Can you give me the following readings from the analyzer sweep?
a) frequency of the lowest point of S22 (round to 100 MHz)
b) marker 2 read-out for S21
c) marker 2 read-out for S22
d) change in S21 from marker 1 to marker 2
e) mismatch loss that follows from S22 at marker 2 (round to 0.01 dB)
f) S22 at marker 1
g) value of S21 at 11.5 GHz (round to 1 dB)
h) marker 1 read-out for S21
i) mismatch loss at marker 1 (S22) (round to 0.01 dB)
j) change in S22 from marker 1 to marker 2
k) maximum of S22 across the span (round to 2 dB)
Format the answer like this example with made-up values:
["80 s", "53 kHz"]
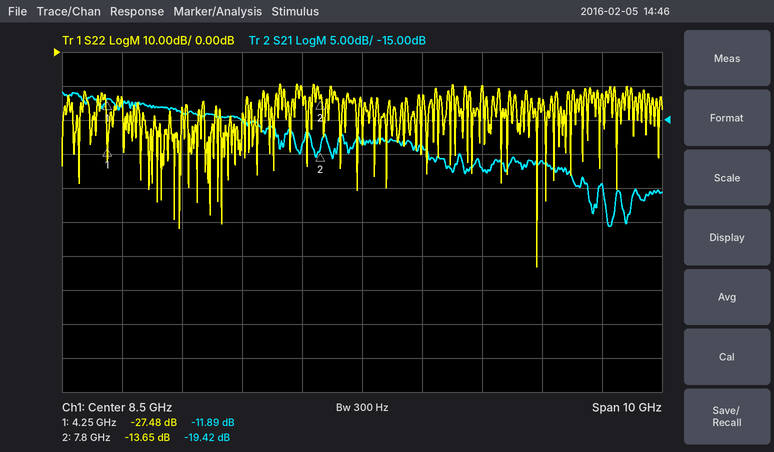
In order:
["11.4 GHz", "-19.42 dB", "-13.65 dB", "-7.53 dB", "0.19 dB", "-27.48 dB", "-21 dB", "-11.89 dB", "0.01 dB", "13.83 dB", "-10 dB"]
